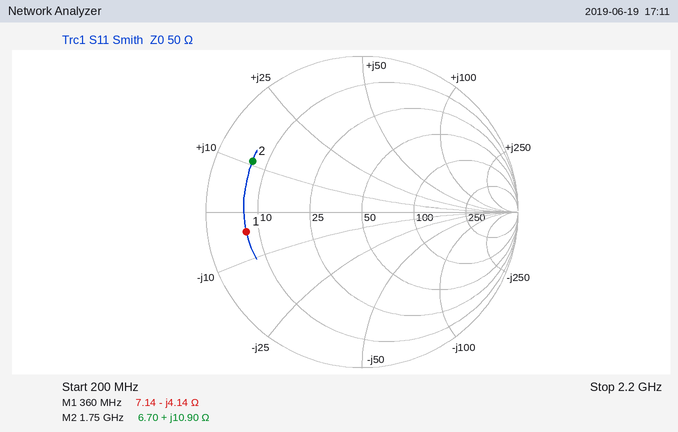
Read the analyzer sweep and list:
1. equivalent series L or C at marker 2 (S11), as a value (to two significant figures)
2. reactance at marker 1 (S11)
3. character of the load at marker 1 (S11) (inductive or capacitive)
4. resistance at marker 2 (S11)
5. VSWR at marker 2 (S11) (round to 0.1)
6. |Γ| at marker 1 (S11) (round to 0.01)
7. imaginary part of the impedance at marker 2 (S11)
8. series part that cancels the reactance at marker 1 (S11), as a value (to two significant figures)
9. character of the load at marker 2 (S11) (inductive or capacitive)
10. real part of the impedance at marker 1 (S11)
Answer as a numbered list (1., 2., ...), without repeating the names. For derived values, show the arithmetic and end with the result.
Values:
1. L = 10.9 Ω/(2π × 1.75 GHz) ≈ 991 pH, so 990 pH to two significant figures
2. -4.14 Ω
3. capacitive
4. 6.70 Ω
5. 7.8
6. 0.75
7. +10.90 Ω
8. L = 4.14 Ω/(2π × 360 MHz) ≈ 1.8 nH
9. inductive
10. 7.14 Ω
